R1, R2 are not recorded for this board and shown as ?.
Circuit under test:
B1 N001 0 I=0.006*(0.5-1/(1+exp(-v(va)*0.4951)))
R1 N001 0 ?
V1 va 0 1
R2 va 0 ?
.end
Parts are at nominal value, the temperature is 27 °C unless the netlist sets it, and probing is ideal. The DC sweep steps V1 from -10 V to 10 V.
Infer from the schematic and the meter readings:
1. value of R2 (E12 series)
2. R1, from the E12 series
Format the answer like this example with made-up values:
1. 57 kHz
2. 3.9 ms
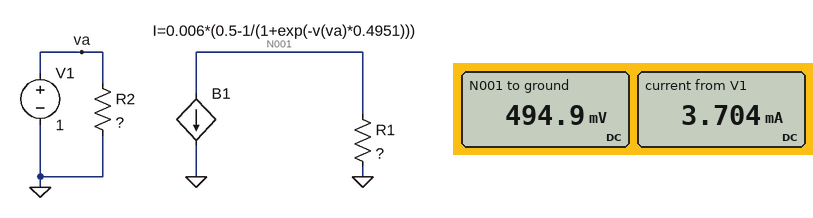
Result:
1. 270 Ω
2. 680 Ω
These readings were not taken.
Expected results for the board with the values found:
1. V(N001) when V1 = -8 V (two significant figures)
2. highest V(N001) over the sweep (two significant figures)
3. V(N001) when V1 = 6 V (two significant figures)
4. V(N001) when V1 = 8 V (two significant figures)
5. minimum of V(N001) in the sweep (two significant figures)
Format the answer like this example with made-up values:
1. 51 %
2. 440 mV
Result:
1. -2.0 V
2. 2.0 V
3. 1.8 V
4. 2.0 V
5. -2.0 V
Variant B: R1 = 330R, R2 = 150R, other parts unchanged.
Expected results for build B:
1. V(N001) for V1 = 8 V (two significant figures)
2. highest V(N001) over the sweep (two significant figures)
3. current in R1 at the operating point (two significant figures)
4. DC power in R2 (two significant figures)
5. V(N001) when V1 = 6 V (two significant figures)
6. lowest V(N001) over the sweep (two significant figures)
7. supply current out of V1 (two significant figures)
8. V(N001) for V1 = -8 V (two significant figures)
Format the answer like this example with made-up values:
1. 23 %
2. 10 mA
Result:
1. 950 mV
2. 980 mV
3. 730 µA
4. 6.7 mW
5. 890 mV
6. -980 mV
7. 6.7 mA
8. -950 mV
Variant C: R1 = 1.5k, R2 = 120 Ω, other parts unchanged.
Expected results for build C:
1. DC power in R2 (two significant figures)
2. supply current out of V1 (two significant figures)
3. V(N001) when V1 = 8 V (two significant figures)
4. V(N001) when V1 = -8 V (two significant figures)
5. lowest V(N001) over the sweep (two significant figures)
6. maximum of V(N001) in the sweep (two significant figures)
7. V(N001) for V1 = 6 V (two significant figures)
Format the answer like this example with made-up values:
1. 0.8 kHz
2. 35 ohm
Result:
1. 8.3 mW
2. 8.3 mA
3. 4.3 V
4. -4.3 V
5. -4.4 V
6. 4.4 V
7. 4.1 V
